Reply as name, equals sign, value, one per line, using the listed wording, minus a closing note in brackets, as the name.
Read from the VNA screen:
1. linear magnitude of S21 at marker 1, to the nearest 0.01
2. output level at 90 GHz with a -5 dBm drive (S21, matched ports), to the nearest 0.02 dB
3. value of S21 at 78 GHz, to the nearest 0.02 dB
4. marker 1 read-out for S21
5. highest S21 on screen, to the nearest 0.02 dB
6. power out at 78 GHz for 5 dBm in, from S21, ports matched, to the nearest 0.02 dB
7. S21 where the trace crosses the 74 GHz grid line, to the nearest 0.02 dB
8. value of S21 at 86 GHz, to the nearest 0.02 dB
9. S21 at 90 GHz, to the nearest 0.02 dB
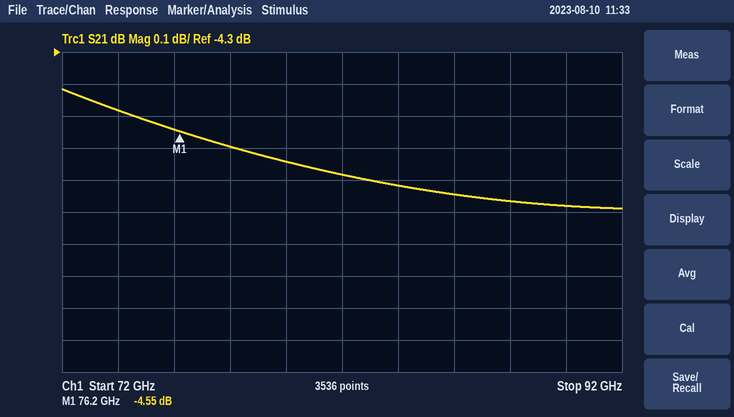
linear magnitude of S21 at marker 1, to the nearest 0.01 = 0.59
output level at 90 GHz with a -5 dBm drive (S21, matched ports), to the nearest 0.02 dB = -9.78 dBm
value of S21 at 78 GHz, to the nearest 0.02 dB = -4.60 dB
marker 1 read-out for S21 = -4.55 dB
highest S21 on screen, to the nearest 0.02 dB = -4.42 dB
power out at 78 GHz for 5 dBm in, from S21, ports matched, to the nearest 0.02 dB = 0.40 dBm
S21 where the trace crosses the 74 GHz grid line, to the nearest 0.02 dB = -4.48 dB
value of S21 at 86 GHz, to the nearest 0.02 dB = -4.74 dB
S21 at 90 GHz, to the nearest 0.02 dB = -4.78 dB
